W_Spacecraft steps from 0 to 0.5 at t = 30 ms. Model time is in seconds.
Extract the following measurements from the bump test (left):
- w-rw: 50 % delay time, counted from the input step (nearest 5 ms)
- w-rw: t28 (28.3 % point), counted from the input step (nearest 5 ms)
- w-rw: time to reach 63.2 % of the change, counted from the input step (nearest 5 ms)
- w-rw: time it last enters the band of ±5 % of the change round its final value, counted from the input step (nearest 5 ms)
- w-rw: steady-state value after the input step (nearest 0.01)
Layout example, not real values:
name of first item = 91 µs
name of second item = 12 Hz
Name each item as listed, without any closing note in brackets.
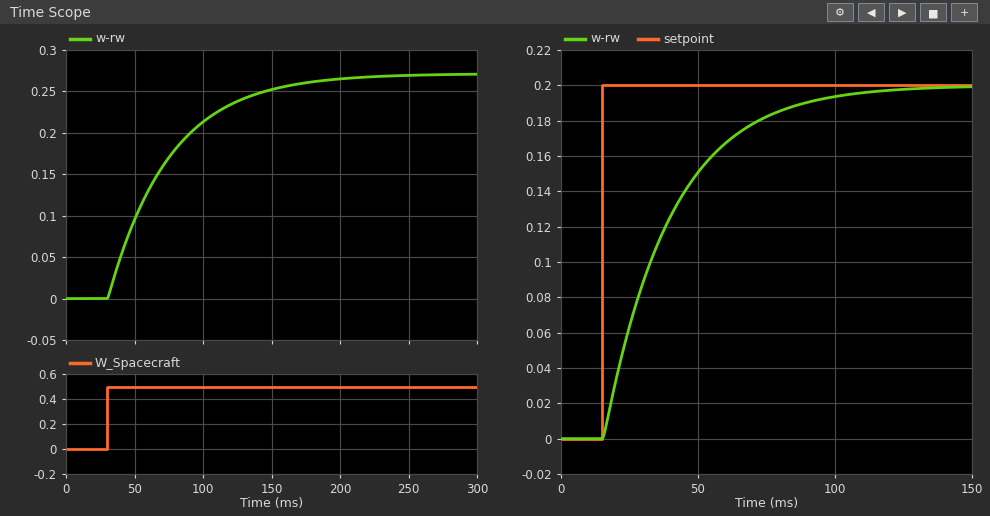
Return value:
w-rw: 50 % delay time, counted from the input step = 30 ms
w-rw: t28 (28.3 % point), counted from the input step = 15 ms
w-rw: time to reach 63.2 % of the change, counted from the input step = 45 ms
w-rw: time it last enters the band of ±5 % of the change round its final value, counted from the input step = 135 ms
w-rw: steady-state value after the input step = 0.27
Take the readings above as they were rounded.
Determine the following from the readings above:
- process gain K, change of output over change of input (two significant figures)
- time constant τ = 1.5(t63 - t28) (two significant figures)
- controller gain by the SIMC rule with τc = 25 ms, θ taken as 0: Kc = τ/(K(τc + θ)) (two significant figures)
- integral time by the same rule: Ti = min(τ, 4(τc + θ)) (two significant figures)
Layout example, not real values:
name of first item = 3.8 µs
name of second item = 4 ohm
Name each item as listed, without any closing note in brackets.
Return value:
process gain K, change of output over change of input = 0.54
time constant τ = 1.5(t63 - t28) = 45 ms
controller gain by the SIMC rule with τc = 25 ms, θ taken as 0: Kc = τ/(K(τc + θ)) = 3.3
integral time by the same rule: Ti = min(τ, 4(τc + θ)) = 45 ms
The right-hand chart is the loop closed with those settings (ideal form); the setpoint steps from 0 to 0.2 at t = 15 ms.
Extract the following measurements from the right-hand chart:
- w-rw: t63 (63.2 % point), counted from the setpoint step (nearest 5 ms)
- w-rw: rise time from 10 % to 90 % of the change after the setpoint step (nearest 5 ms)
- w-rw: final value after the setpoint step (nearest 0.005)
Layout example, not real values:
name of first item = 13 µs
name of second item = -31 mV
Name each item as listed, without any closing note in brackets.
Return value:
w-rw: t63 (63.2 % point), counted from the setpoint step = 25 ms
w-rw: rise time from 10 % to 90 % of the change after the setpoint step = 55 ms
w-rw: final value after the setpoint step = 0.200
